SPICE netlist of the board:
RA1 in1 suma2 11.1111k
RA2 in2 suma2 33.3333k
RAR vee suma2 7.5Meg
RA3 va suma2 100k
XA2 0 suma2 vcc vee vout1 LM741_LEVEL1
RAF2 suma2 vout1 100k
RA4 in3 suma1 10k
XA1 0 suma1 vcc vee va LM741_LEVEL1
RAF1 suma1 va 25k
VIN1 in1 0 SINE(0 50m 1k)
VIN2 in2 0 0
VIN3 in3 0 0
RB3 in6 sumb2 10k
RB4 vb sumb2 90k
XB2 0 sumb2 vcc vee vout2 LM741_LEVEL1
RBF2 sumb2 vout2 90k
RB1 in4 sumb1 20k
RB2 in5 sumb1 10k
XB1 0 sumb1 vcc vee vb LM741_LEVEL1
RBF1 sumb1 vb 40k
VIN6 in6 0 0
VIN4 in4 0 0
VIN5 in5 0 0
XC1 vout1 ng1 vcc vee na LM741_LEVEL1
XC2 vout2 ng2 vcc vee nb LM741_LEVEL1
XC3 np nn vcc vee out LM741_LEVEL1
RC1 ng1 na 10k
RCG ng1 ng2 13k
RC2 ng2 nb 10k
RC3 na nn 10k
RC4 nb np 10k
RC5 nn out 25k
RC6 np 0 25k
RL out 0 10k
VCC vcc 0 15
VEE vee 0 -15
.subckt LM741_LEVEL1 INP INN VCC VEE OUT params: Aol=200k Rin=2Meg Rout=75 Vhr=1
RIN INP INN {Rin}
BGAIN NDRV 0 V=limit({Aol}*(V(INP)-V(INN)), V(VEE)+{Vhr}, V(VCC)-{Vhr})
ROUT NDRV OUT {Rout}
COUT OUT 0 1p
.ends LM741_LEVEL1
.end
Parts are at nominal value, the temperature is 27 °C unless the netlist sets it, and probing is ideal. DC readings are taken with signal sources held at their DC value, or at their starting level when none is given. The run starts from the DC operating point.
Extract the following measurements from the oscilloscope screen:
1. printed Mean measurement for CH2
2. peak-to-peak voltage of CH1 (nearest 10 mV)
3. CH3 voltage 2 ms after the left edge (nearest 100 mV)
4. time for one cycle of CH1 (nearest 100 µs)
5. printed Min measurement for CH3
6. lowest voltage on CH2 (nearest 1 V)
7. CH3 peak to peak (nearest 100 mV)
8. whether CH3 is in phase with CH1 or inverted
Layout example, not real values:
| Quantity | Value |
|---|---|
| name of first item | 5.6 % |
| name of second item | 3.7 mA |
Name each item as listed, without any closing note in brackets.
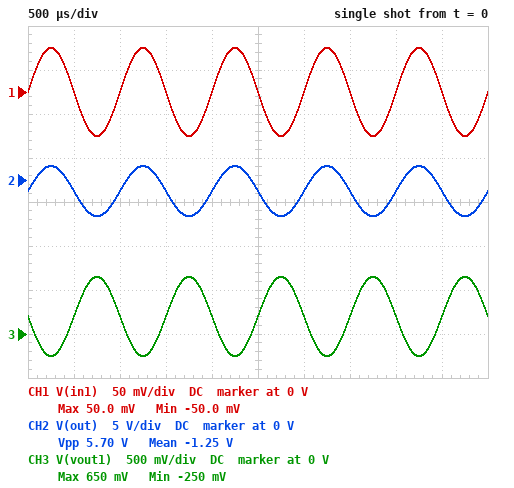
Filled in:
| Quantity | Value |
|---|---|
| printed Mean measurement for CH2 | -1.25 V |
| peak-to-peak voltage of CH1 | 100 mV |
| CH3 voltage 2 ms after the left edge | 200 mV |
| time for one cycle of CH1 | 1.0 ms |
| printed Min measurement for CH3 | -250 mV |
| lowest voltage on CH2 | -4 V |
| CH3 peak to peak | 900 mV |
| whether CH3 is in phase with CH1 or inverted | inverted |
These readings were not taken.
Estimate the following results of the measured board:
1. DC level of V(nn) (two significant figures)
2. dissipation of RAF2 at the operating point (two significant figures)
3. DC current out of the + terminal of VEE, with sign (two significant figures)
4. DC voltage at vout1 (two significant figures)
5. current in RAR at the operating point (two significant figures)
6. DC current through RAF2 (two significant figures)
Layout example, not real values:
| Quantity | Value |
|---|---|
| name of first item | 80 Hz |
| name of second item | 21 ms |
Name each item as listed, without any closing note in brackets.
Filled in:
| Quantity | Value |
|---|---|
| DC level of V(nn) | -110 mV |
| dissipation of RAF2 at the operating point | 400 nW |
| DC current out of the + terminal of VEE, with sign | -2.0 µA |
| DC voltage at vout1 | 200 mV |
| current in RAR at the operating point | 2.0 µA |
| DC current through RAF2 | 2.0 µA |
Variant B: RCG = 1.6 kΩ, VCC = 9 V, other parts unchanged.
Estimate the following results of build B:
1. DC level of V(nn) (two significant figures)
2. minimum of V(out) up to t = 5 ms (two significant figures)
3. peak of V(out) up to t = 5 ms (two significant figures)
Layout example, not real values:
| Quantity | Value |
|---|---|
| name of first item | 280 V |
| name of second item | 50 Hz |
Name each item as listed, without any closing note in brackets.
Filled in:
| Quantity | Value |
|---|---|
| DC level of V(nn) | -890 mV |
| minimum of V(out) up to t = 5 ms | -14 V |
| peak of V(out) up to t = 5 ms | 7.9 V |
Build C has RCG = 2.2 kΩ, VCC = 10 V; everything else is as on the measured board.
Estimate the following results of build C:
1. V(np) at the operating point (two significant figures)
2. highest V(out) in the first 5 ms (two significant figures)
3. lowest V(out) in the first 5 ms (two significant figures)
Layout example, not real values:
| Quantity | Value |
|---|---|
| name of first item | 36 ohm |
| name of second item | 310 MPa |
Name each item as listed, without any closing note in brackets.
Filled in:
| Quantity | Value |
|---|---|
| V(np) at the operating point | -650 mV |
| highest V(out) in the first 5 ms | 6.3 V |
| lowest V(out) in the first 5 ms | -14 V |
